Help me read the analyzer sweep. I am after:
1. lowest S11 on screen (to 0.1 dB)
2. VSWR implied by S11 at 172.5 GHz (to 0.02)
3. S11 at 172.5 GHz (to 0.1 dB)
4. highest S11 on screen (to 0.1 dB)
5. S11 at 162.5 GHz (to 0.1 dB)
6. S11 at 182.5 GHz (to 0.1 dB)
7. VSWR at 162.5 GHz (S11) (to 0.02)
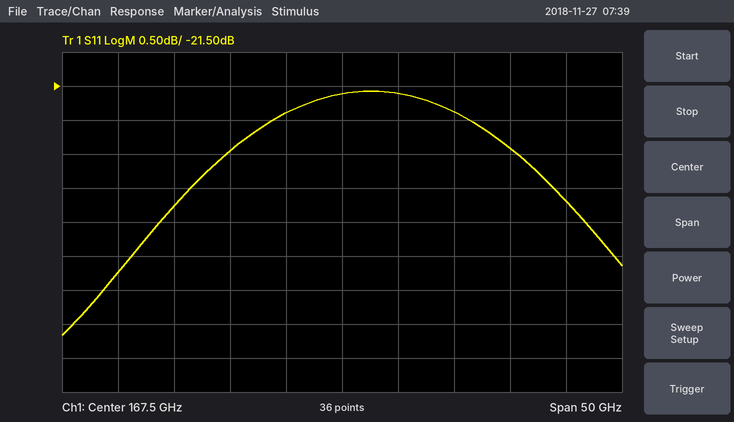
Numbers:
-25.2 dB
1.18
-21.6 dB
-21.6 dB
-21.9 dB
-22.4 dB
1.18
